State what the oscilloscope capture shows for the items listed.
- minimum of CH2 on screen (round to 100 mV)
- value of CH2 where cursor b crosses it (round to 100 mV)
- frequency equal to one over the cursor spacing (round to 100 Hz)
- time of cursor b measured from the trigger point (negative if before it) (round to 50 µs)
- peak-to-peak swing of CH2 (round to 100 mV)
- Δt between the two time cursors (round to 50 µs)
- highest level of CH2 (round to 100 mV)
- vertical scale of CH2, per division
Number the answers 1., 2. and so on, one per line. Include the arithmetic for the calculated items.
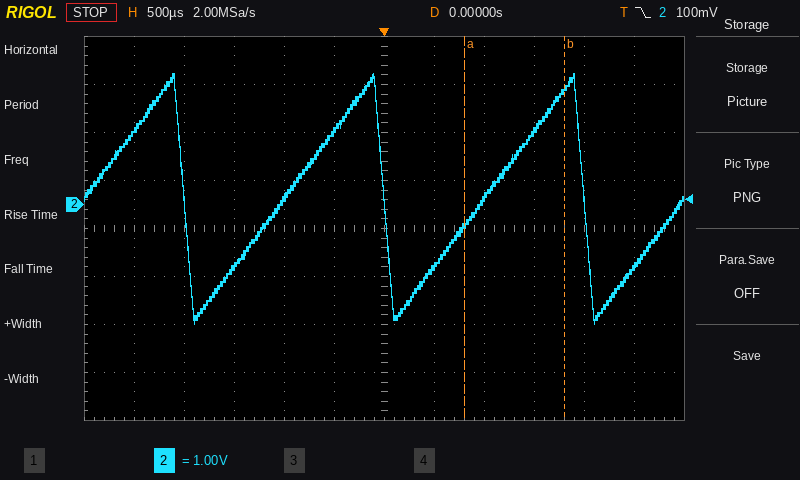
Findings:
1. -2.5 V
2. 2.4 V
3. 1 / 1.00 ms ≈ 1.0 kHz
4. +1.80 ms
5. 2.7 V − (-2.5 V) = 5.2 V
6. 1.00 ms
7. 2.7 V
8. 1 V
